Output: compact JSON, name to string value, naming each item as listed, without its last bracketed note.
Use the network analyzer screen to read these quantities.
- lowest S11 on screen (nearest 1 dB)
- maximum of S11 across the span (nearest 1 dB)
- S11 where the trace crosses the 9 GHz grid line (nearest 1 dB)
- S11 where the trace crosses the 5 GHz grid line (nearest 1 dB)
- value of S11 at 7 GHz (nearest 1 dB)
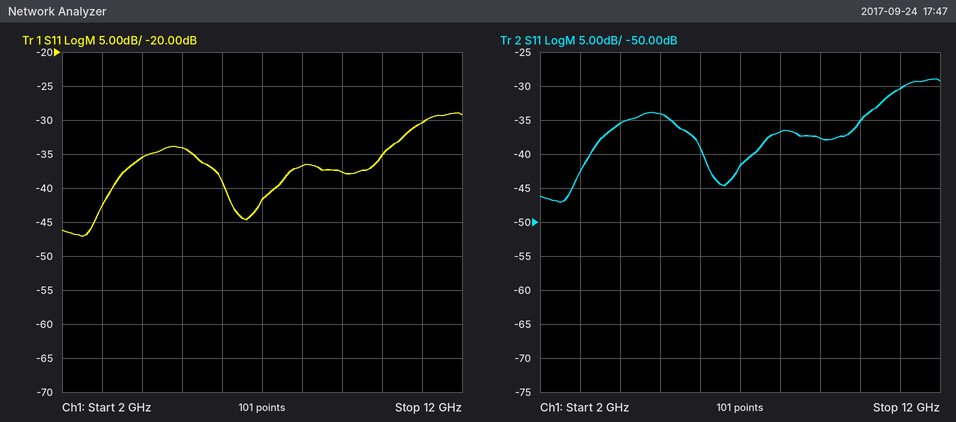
{"lowest S11 on screen": "-47 dB", "maximum of S11 across the span": "-29 dB", "S11 where the trace crosses the 9 GHz grid line": "-38 dB", "S11 where the trace crosses the 5 GHz grid line": "-34 dB", "value of S11 at 7 GHz": "-42 dB"}
